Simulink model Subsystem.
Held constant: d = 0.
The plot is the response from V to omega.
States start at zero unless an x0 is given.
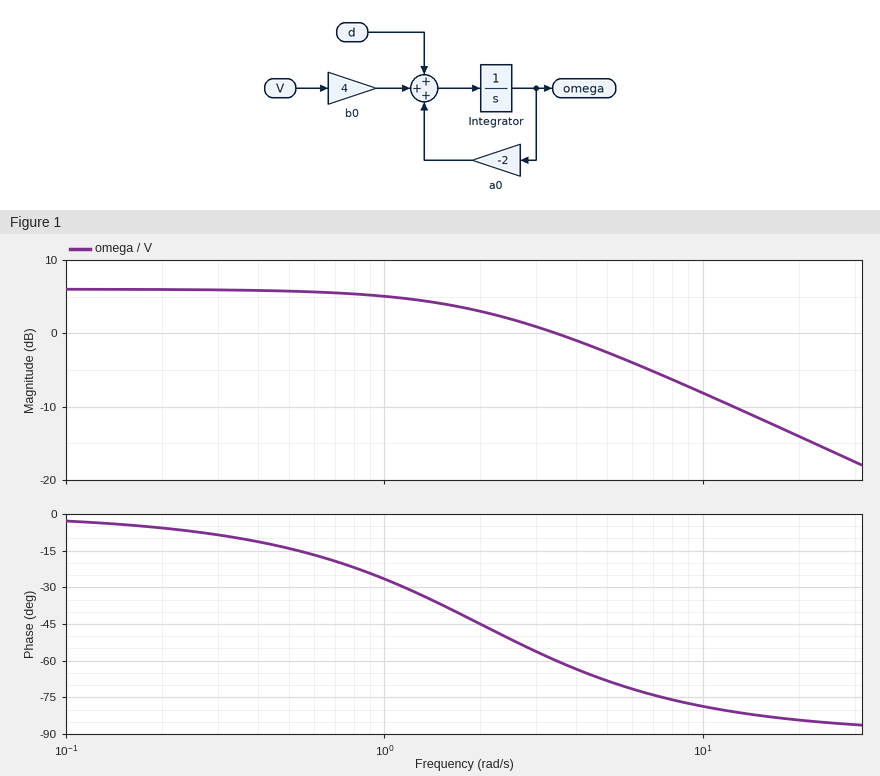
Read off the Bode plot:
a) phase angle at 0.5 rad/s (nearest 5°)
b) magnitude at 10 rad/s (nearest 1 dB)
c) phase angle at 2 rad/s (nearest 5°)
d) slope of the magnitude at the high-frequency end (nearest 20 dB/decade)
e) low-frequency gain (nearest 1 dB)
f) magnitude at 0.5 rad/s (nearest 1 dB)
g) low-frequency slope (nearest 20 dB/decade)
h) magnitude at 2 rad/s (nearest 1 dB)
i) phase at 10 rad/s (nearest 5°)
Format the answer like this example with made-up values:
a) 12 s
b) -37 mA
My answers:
a) -15°
b) -8 dB
c) -45°
d) -20 dB/decade
e) 6 dB
f) 6 dB
g) 0 dB/decade
h) 3 dB
i) -80°
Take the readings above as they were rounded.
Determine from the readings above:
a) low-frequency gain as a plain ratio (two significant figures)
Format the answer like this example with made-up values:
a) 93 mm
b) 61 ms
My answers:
a) 2.0
